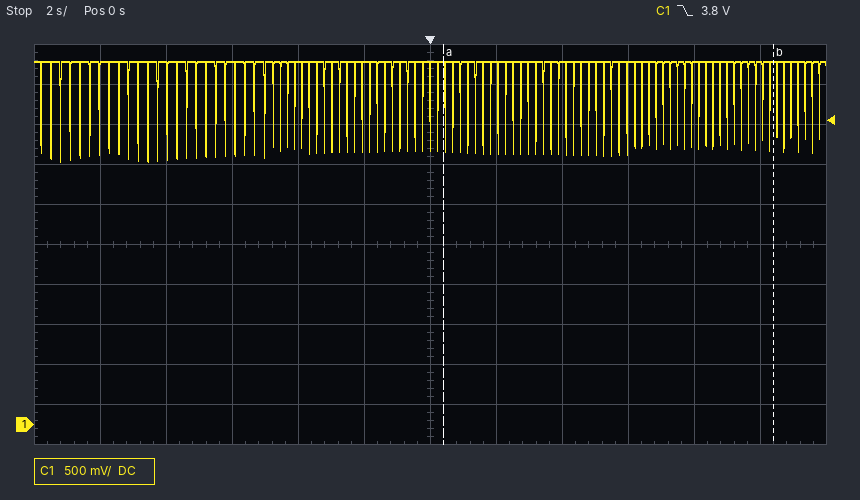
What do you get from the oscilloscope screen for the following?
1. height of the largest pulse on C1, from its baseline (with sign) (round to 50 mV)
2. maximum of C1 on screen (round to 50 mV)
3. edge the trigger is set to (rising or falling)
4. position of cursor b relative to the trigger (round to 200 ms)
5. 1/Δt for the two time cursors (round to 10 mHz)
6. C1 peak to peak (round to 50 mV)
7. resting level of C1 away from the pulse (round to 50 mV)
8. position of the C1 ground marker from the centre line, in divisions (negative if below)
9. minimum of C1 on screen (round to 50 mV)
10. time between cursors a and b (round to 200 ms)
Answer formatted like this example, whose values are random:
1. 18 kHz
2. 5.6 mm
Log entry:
1. -1.25 V
2. 4.55 V
3. falling
4. +10.4 s
5. 100 mHz
6. 1.25 V
7. 4.55 V
8. -4.5 div
9. 3.30 V
10. 10.0 s
